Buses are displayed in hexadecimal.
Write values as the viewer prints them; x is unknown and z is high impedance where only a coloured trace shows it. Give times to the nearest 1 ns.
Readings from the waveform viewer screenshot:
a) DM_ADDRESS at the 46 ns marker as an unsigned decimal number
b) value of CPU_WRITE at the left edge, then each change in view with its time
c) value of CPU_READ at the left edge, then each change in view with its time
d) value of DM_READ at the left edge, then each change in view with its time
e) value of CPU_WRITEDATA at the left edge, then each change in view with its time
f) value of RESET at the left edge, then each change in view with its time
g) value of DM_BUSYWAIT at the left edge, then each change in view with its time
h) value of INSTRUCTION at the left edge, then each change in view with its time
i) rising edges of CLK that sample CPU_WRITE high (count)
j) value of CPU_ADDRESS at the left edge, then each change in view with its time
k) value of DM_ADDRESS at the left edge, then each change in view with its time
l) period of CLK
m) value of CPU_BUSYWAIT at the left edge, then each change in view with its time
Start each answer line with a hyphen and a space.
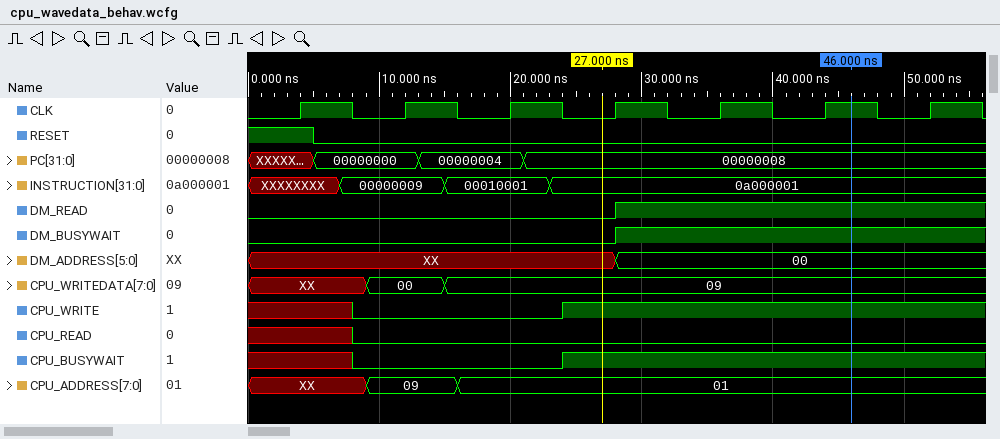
- 0
- x, 0 at 8 ns, 1 at 24 ns
- x, 0 at 8 ns
- 0, 1 at 28 ns
- XX, 00 at 9 ns, 09 at 15 ns
- 1, 0 at 5 ns
- 0, 1 at 28 ns
- XXXXXXXX, 00000009 at 7 ns, 00010001 at 15 ns, 0a000001 at 23 ns
- 4
- XX, 09 at 9 ns, 01 at 16 ns
- XX, 00 at 28 ns
- 8 ns
- x, 0 at 8 ns, 1 at 24 ns
